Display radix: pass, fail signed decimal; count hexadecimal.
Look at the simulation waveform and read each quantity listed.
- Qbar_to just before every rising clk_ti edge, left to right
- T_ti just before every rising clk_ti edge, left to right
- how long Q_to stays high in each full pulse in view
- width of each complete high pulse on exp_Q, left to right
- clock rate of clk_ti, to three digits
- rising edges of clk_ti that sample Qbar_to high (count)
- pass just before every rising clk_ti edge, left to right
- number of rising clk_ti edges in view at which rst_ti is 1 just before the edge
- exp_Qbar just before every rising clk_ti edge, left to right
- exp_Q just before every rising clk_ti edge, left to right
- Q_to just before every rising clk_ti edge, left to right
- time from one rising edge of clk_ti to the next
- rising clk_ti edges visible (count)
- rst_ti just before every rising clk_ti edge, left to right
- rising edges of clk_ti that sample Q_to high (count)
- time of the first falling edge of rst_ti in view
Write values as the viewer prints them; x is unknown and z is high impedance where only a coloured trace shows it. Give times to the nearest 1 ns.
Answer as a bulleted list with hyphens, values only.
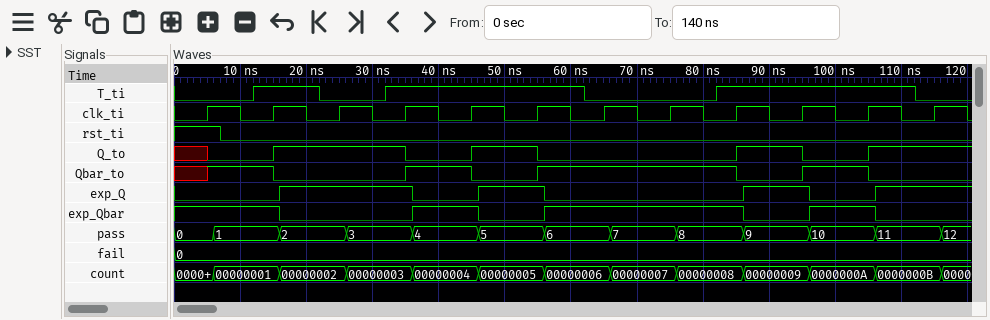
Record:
- x 1 0 0 1 0 1 1 1 0 1 0
- 0 1 0 1 1 1 0 0 1 1 1 0
- 20 ns, 10 ns, 10 ns
- 20 ns, 10 ns, 10 ns
- 100 MHz
- 6
- 0, 1, 2, 3, 4, 5, 6, 7, 8, 9, 10, 11
- 1
- 1 1 0 0 1 0 1 1 1 0 1 0
- 0 0 1 1 0 1 0 0 0 1 0 1
- x 0 1 1 0 1 0 0 0 1 0 1
- 10 ns
- 12
- 1 0 0 0 0 0 0 0 0 0 0 0
- 5
- 7 ns
